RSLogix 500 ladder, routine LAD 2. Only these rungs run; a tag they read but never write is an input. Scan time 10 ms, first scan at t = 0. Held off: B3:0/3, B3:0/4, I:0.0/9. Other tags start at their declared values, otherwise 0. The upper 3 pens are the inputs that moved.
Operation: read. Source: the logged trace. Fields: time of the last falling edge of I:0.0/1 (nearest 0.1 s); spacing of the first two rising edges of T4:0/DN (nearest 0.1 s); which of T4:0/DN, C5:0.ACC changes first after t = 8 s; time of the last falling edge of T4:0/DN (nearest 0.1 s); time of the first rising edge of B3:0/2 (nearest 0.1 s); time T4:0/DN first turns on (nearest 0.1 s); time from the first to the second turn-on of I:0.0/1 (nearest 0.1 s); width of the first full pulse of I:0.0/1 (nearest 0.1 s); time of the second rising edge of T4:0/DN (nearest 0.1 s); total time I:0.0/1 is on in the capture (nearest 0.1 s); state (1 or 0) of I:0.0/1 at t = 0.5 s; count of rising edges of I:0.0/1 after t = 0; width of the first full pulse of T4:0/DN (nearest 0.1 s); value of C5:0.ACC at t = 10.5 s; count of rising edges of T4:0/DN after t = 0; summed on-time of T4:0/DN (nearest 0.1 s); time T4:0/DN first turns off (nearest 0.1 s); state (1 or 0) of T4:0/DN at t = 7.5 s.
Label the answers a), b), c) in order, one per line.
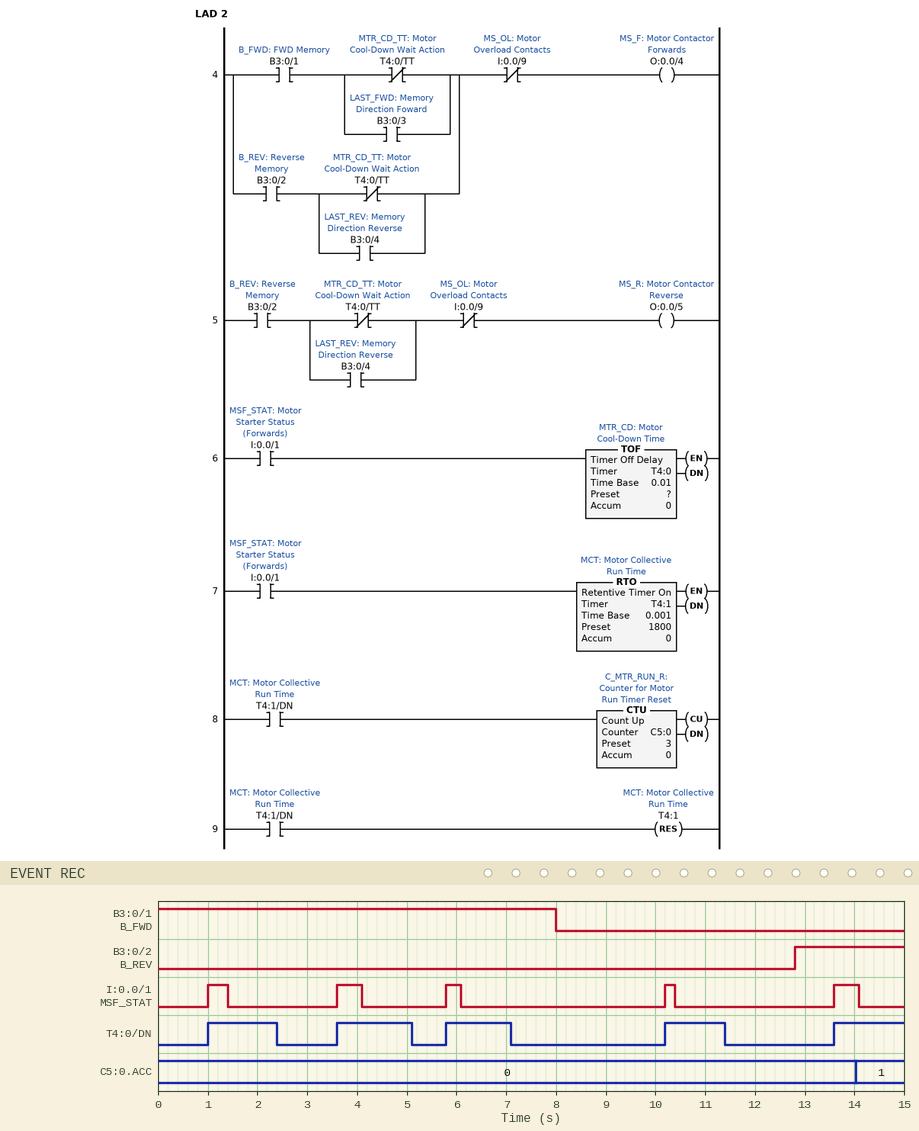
a) 14.1 s
b) 2.6 s
c) T4:0/DN
d) 11.4 s
e) 12.8 s
f) 1.0 s
g) 2.6 s
h) 0.4 s
i) 3.6 s
j) 1.9 s
k) 0
l) 5
m) 1.4 s
n) 0
o) 5
p) 6.8 s
q) 2.4 s
r) 0
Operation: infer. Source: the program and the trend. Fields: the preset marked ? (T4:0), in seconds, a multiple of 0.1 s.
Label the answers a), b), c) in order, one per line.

a) 1.0 s
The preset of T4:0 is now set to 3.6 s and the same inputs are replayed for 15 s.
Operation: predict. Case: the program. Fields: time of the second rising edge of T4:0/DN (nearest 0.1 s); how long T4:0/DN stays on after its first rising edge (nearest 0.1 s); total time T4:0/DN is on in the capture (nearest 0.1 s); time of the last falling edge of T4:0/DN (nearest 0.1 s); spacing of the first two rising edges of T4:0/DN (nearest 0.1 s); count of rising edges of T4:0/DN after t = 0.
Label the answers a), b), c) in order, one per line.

a) 10.2 s
b) 8.7 s
c) 13.5 s
d) 9.7 s
e) 9.2 s
f) 2
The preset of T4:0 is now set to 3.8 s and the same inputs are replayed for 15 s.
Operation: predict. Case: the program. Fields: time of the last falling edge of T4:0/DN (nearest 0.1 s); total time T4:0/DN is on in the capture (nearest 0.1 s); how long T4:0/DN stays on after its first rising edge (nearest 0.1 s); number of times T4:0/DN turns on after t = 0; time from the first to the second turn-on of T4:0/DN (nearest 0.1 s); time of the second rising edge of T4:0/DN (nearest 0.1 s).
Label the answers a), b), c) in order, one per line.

a) 9.9 s
b) 13.7 s
c) 8.9 s
d) 2
e) 9.2 s
f) 10.2 s
